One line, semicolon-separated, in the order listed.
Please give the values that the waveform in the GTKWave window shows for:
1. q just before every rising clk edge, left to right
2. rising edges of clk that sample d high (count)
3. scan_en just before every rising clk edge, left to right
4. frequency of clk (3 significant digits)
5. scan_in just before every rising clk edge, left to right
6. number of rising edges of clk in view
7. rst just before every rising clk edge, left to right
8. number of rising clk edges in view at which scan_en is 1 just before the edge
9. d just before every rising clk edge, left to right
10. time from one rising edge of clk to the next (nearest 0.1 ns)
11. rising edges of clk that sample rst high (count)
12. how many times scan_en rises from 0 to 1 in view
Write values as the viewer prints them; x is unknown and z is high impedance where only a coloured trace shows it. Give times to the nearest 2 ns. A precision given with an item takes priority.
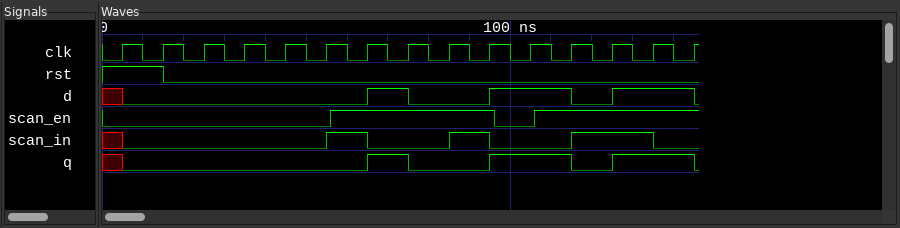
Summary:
x 0 0 0 0 0 0 1 0 0 1 1 0 1 1; 5; 0 0 0 0 0 0 1 1 1 1 0 1 1 1 1; 100 MHz; x 0 0 0 0 0 1 0 0 1 0 0 1 1 0; 15; 1 1 0 0 0 0 0 0 0 0 0 0 0 0 0; 8; x 0 0 0 0 0 0 1 0 0 1 1 0 1 1; 10 ns; 2; 2
